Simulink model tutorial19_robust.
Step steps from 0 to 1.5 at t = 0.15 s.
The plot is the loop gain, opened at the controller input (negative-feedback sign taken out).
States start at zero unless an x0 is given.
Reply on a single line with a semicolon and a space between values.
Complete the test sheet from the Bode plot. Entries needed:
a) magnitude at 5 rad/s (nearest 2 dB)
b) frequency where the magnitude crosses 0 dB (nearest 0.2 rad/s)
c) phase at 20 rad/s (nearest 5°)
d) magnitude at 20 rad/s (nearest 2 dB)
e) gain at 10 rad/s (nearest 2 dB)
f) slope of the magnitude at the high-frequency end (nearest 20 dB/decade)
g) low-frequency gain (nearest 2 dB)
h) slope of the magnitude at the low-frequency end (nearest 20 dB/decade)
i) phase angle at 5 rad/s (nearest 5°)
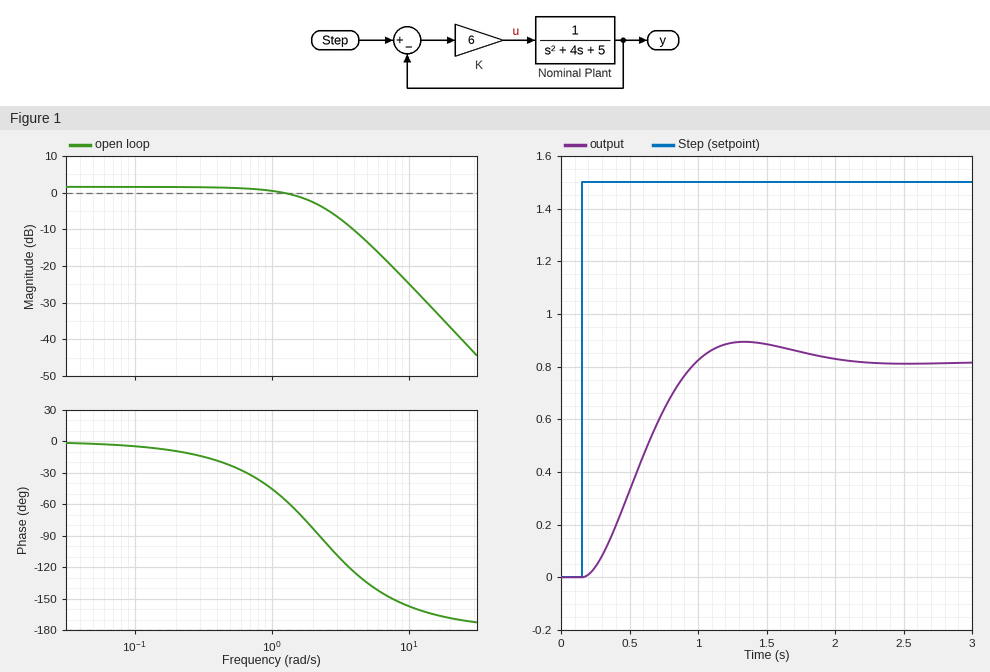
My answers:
-14 dB; 1.2 rad/s; -170°; -36 dB; -24 dB; -40 dB/decade; 2 dB; 0 dB/decade; -135°
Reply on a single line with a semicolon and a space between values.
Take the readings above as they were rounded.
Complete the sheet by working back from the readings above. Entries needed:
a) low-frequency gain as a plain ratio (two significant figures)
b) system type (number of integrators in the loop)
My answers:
1.3; 0
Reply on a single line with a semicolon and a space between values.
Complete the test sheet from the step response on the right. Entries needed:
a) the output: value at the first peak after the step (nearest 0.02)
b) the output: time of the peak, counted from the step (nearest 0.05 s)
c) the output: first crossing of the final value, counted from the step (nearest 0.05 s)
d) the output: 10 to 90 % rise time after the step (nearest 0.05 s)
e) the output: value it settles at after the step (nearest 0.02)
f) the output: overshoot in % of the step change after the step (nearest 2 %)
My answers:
0.90; 1.20 s; 0.85 s; 0.55 s; 0.82; 10 %
